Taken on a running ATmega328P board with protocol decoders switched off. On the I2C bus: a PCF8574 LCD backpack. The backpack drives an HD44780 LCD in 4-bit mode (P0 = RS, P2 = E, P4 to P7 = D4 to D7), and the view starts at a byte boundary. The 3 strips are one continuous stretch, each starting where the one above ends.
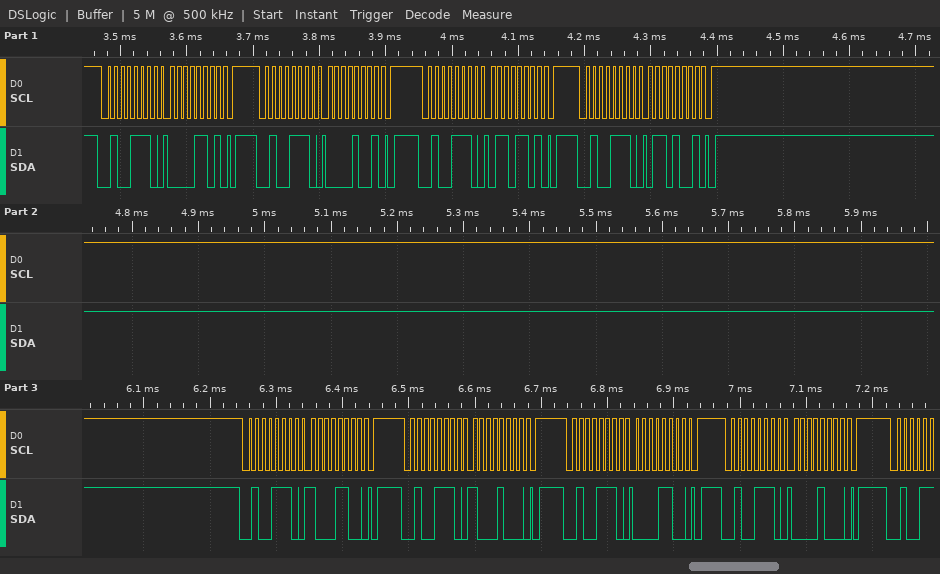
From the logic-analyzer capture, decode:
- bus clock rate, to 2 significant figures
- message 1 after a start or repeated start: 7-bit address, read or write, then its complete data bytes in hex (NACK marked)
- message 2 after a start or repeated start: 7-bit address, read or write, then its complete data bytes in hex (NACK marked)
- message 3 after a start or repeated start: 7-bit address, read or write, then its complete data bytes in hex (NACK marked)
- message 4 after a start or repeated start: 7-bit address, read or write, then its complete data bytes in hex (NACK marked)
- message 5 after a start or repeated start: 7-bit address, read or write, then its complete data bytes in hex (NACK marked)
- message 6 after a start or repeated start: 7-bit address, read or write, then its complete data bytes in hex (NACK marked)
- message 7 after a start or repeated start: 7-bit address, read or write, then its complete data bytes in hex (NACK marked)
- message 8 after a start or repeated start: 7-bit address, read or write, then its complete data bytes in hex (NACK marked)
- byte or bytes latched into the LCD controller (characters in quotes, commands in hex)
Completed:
100 kHz
0x27 write: 0D
0x27 write: 09
0x27 write: 6D
0x27 write: 69
0x27 write: 8C
0x27 write: 88
0x27 write: 0C
0x27 write: 08
data 0x06 0x80
